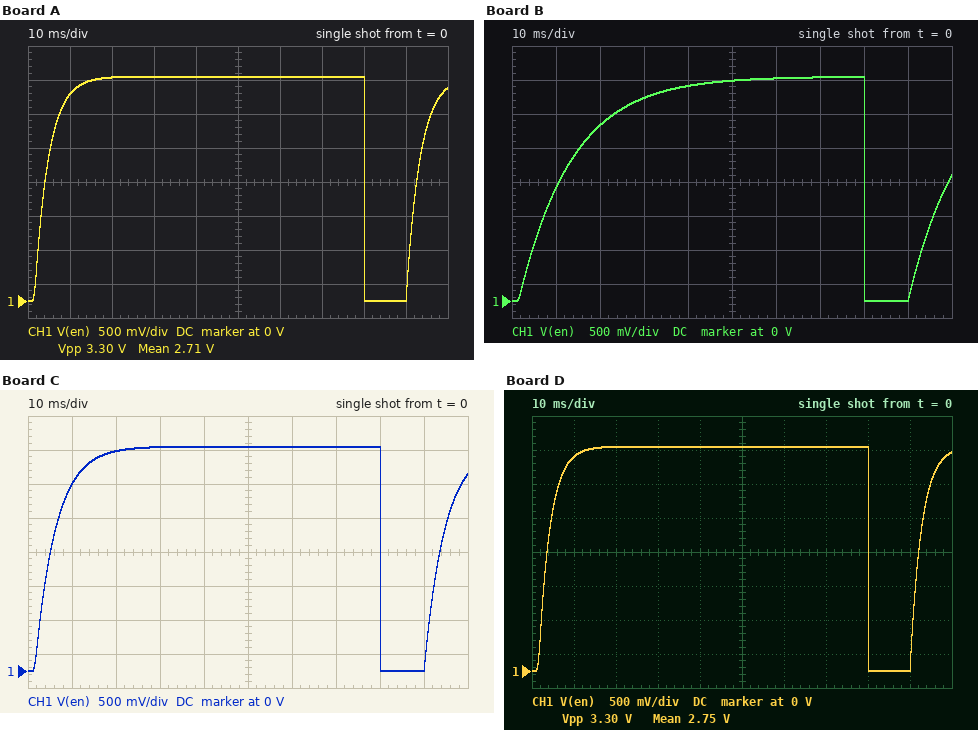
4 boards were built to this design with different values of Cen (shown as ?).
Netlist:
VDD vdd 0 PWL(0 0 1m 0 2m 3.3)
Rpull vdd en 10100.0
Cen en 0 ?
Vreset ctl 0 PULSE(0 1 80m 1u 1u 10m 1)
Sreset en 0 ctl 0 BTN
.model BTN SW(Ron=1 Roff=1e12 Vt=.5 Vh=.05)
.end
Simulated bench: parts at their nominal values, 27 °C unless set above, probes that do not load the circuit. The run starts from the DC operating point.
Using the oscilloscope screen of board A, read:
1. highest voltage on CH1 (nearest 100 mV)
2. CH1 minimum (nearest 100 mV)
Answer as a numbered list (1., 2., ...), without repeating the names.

1. 3.3 V
2. 0 V
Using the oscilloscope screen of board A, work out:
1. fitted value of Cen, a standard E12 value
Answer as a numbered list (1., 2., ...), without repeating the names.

1. 330 nF
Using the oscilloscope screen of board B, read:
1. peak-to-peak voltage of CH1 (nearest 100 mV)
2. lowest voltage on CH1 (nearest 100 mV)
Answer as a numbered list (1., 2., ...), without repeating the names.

1. 3.3 V
2. 0 V
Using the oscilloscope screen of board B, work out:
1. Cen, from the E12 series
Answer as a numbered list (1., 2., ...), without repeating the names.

1. 1.2 µF
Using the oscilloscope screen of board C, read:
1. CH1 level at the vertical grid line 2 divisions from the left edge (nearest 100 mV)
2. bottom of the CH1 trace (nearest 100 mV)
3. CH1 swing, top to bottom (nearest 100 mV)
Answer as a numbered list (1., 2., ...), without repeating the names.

1. 3.2 V
2. 0 V
3. 3.3 V
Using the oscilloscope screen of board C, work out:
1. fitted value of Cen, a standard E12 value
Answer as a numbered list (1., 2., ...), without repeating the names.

1. 470 nF
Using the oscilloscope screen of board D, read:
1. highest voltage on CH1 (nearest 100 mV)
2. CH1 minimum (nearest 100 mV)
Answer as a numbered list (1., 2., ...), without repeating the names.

1. 3.3 V
2. 0 V
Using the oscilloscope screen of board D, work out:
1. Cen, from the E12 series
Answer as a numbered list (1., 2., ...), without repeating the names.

1. 270 nF
